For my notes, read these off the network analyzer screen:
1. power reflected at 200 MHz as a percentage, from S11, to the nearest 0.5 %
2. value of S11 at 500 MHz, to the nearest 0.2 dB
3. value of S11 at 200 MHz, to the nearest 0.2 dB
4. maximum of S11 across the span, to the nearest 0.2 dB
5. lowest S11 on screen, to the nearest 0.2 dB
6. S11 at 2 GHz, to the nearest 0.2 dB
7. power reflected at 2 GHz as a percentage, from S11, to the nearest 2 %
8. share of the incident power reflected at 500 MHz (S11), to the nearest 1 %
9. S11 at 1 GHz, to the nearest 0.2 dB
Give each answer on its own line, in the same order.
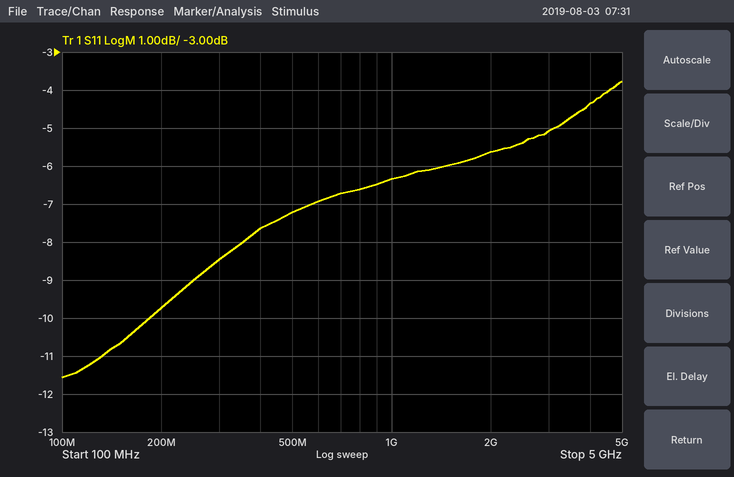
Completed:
10.5 %
-7.2 dB
-9.8 dB
-3.8 dB
-11.6 dB
-5.6 dB
28 %
19 %
-6.4 dB
